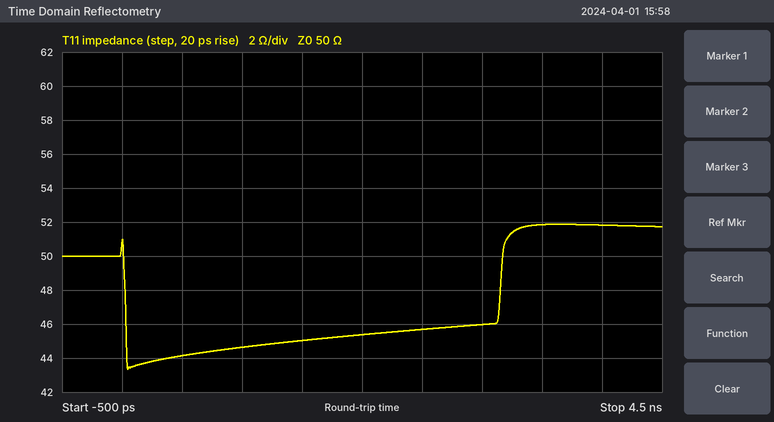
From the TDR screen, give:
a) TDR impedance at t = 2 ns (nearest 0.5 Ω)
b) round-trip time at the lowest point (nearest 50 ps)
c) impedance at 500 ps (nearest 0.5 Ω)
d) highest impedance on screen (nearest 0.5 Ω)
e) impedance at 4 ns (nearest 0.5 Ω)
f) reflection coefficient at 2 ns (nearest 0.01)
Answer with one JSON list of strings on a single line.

["45.5 Ω", "50 ps", "44.0 Ω", "52.0 Ω", "52.0 Ω", "-0.05"]
